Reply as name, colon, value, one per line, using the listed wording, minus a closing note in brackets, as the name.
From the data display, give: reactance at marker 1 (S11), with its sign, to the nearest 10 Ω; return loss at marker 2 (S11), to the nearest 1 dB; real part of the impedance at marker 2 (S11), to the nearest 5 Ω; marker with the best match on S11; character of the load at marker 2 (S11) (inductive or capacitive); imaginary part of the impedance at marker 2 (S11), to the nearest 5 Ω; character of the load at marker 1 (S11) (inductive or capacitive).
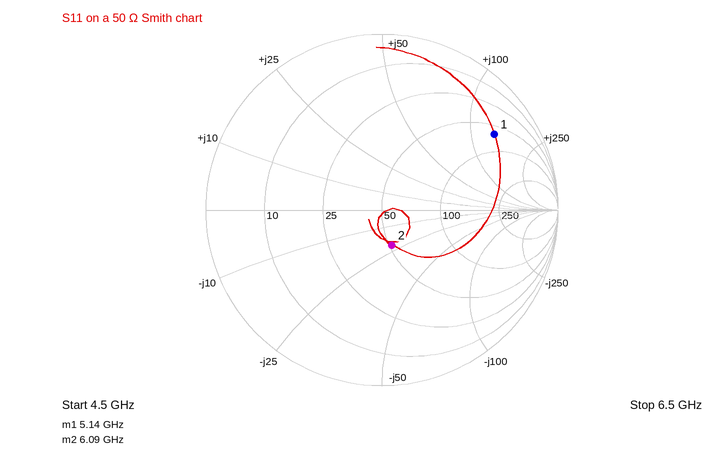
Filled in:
reactance at marker 1 (S11), with its sign, to the nearest 10 Ω: +140 Ω
return loss at marker 2 (S11), to the nearest 1 dB: 14 dB
real part of the impedance at marker 2 (S11), to the nearest 5 Ω: 50 Ω
marker with the best match on S11: marker 2
character of the load at marker 2 (S11): capacitive
imaginary part of the impedance at marker 2 (S11), to the nearest 5 Ω: -20 Ω
character of the load at marker 1 (S11): inductive
